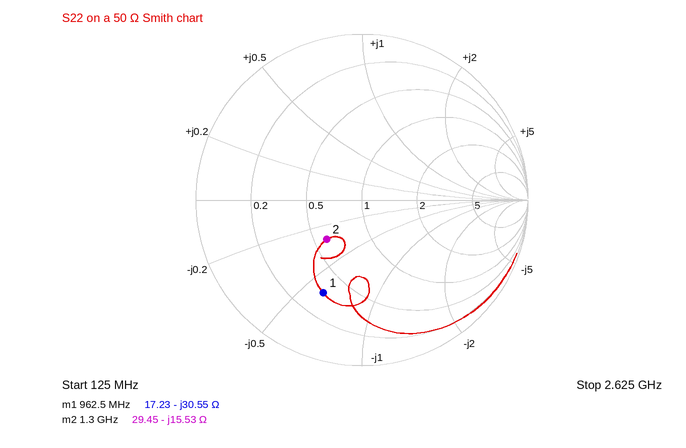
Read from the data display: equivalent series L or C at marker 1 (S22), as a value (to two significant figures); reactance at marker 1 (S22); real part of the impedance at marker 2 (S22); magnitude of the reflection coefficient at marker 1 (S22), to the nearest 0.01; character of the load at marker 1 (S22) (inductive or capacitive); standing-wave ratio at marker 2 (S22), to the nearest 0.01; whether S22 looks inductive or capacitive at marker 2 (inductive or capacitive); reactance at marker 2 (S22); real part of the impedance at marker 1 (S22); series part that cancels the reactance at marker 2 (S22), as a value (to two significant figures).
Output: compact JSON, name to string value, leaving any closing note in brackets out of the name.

{"equivalent series L or C at marker 1 (S22), as a value": "5.4 pF", "reactance at marker 1": "-30.55 Ω", "real part of the impedance at marker 2": "29.45 Ω", "magnitude of the reflection coefficient at marker 1 (S22), to the nearest 0.01": "0.61", "character of the load at marker 1 (S22)": "capacitive", "standing-wave ratio at marker 2 (S22), to the nearest 0.01": "1.93", "whether S22 looks inductive or capacitive at marker 2": "capacitive", "reactance at marker 2": "-15.53 Ω", "real part of the impedance at marker 1": "17.23 Ω", "series part that cancels the reactance at marker 2 (S22), as a value": "1.9 nH"}
